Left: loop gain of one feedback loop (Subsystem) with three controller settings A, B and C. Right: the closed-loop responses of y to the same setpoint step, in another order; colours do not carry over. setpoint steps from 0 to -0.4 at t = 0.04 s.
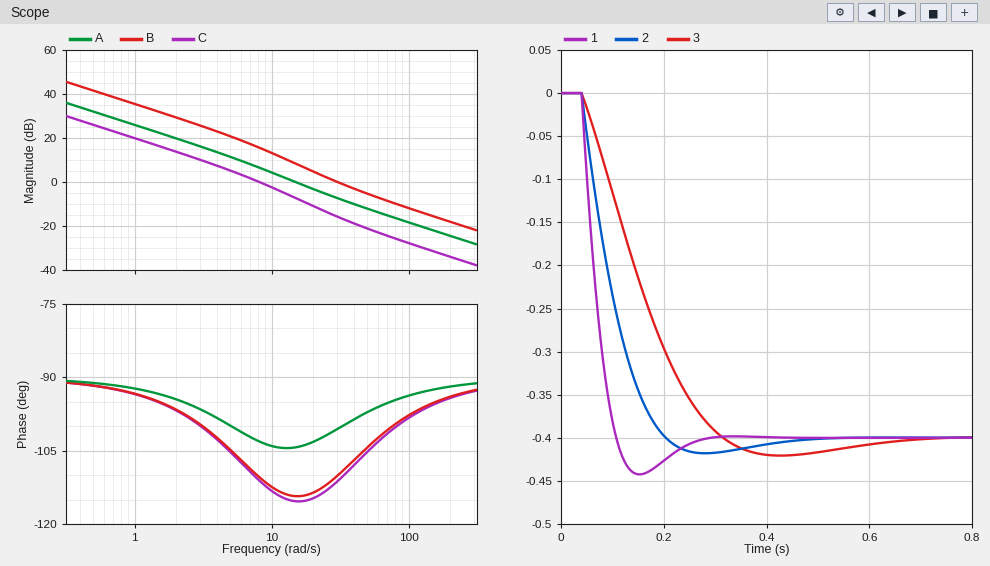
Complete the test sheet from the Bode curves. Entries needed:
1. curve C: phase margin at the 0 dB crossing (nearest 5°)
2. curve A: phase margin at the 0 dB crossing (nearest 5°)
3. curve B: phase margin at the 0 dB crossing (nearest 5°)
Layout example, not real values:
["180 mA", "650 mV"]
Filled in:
["70°", "75°", "70°"]
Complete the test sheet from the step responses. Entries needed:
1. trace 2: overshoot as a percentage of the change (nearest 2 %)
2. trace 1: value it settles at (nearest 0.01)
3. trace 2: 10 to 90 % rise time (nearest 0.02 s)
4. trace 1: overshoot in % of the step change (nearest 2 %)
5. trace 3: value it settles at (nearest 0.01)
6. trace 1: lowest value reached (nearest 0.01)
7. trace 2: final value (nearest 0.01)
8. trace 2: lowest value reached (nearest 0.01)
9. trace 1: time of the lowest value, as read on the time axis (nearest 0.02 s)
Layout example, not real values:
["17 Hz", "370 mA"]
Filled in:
["4 %", "-0.40", "0.12 s", "10 %", "-0.40", "-0.44", "-0.40", "-0.42", "0.16 s"]
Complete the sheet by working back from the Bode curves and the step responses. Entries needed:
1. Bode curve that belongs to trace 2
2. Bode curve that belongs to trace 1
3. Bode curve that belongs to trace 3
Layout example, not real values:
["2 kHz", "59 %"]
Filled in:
["A", "B", "C"]
